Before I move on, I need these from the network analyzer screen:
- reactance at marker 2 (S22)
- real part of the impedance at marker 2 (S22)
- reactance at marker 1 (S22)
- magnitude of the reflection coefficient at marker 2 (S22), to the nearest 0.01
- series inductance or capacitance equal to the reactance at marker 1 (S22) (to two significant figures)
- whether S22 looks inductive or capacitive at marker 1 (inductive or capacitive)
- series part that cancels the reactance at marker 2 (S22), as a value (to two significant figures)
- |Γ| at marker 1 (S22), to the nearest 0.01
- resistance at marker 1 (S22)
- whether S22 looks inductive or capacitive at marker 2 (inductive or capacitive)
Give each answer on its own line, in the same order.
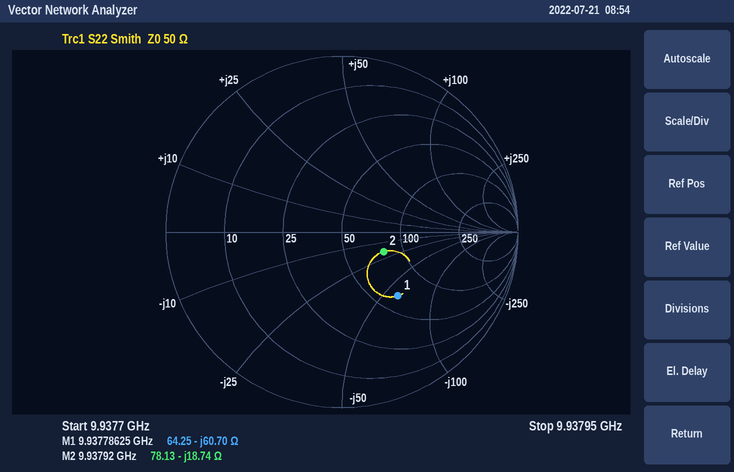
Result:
-18.74 Ω
78.13 Ω
-60.70 Ω
0.26
260 fF
capacitive
300 pH
0.48
64.25 Ω
capacitive
